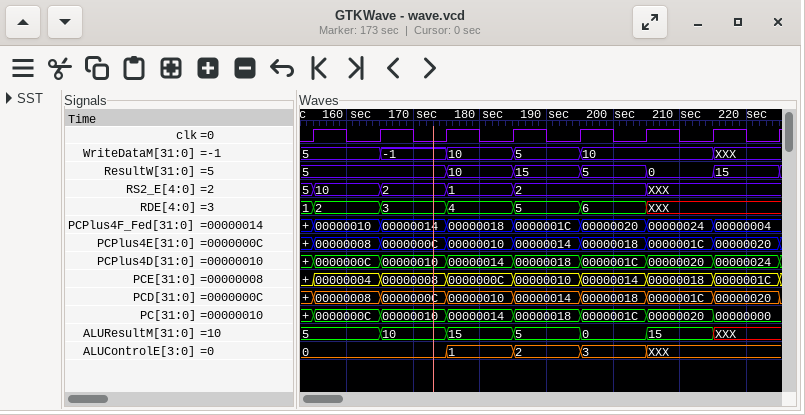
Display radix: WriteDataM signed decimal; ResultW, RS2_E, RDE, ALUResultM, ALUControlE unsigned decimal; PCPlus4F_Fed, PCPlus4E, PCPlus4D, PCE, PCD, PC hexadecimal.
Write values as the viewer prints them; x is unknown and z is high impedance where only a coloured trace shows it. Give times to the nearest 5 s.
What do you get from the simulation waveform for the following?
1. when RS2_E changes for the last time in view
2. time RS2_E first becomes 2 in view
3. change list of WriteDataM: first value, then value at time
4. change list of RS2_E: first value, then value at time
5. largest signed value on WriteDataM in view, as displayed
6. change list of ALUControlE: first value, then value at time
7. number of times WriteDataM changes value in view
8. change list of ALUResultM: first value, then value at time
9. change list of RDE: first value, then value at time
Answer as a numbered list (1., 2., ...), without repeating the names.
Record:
1. 205 s
2. 165 s
3. 5, -1 at 165 s, 10 at 175 s, 5 at 185 s, 10 at 195 s, XXX at 215 s
4. 5, 10 at 155 s, 2 at 165 s, 1 at 175 s, 2 at 185 s, XXX at 205 s
5. 10
6. 0, 1 at 175 s, 2 at 185 s, 3 at 195 s, XXX at 205 s
7. 5
8. 5, 10 at 165 s, 15 at 175 s, 5 at 185 s, 0 at 195 s, 15 at 205 s, XXX at 215 s
9. 1, 2 at 155 s, 3 at 165 s, 4 at 175 s, 5 at 185 s, 6 at 195 s, XXX at 205 s
